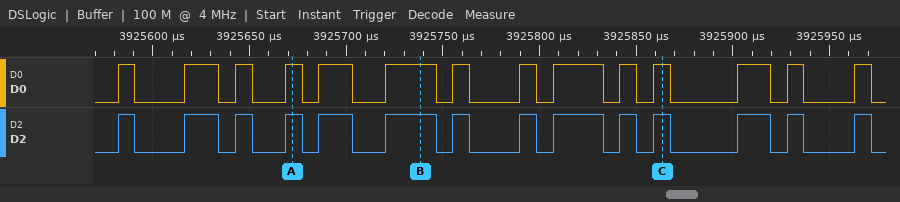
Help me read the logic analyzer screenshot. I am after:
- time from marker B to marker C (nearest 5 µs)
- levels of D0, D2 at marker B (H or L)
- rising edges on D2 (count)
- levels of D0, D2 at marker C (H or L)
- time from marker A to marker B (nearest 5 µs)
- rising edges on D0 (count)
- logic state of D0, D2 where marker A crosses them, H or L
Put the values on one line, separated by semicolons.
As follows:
125 µs; D0=H, D2=H; 14; D0=H, D2=H; 65 µs; 14; D0=H, D2=H
